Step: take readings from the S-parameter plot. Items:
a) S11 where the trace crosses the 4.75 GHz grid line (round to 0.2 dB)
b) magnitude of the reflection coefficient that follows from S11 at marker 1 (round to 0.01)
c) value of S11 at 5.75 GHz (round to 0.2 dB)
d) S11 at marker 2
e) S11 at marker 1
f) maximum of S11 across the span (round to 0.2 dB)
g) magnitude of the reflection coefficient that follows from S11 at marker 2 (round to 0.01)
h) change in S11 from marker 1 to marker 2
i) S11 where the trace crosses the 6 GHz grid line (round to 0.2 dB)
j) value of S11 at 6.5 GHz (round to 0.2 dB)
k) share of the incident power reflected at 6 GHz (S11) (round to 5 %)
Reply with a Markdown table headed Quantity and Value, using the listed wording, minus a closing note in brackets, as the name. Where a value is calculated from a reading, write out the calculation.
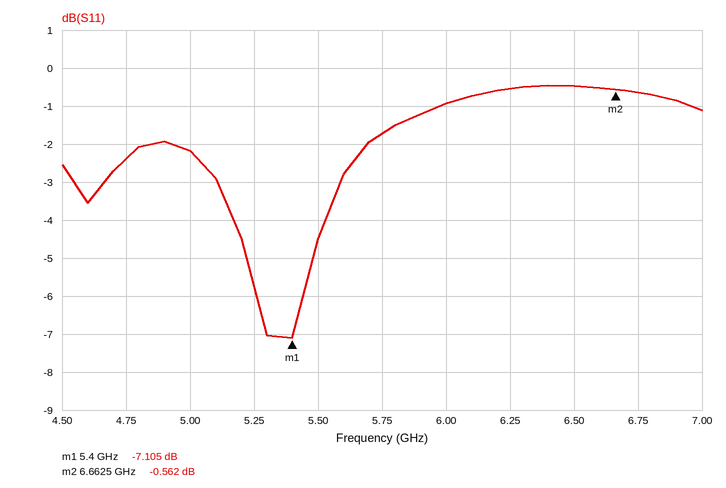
| Quantity | Value |
|---|---|
| S11 where the trace crosses the 4.75 GHz grid line | -2.4 dB |
| magnitude of the reflection coefficient that follows from S11 at marker 1 | 10^(-7.105/20) ≈ 0.44 |
| value of S11 at 5.75 GHz | -1.8 dB |
| S11 at marker 2 | -0.562 dB |
| S11 at marker 1 | -7.105 dB |
| maximum of S11 across the span | -0.4 dB |
| magnitude of the reflection coefficient that follows from S11 at marker 2 | 10^(-0.562/20) ≈ 0.94 |
| change in S11 from marker 1 to marker 2 | -0.562 − (-7.105) = 6.543 dB |
| S11 where the trace crosses the 6 GHz grid line | -1.0 dB |
| value of S11 at 6.5 GHz | -0.4 dB |
| share of the incident power reflected at 6 GHz (S11) | 10^(-1/10) ≈ 79.4 %, so 80 % to the nearest 5 % |
